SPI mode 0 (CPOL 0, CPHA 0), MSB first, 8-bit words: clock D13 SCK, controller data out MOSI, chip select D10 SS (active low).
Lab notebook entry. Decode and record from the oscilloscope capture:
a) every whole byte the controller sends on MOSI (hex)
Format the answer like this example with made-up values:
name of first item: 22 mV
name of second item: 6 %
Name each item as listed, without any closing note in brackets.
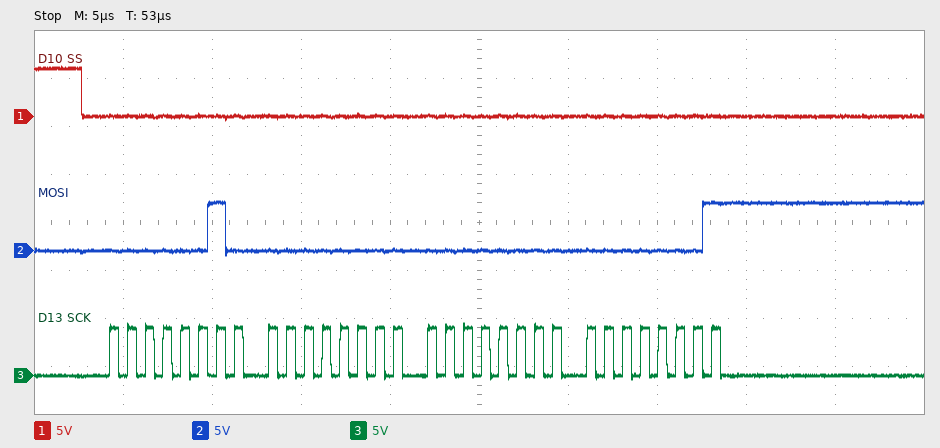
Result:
every whole byte the controller sends on MOSI: 0x02 0x00 0x00 0x01
